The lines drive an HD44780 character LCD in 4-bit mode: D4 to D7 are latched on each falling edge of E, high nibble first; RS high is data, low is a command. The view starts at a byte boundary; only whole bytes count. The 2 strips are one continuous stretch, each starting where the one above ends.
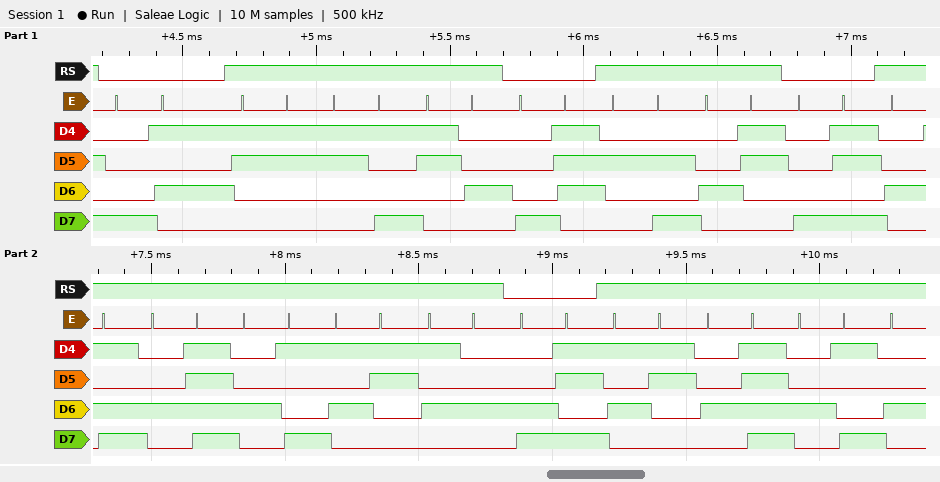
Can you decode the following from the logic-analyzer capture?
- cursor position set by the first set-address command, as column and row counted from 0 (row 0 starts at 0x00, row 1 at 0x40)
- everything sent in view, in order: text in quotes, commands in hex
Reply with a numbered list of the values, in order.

1. column 5, row 0
2. 0x85 "394" 0x87 "*C" 0x8B "MOIST" 0xCB "SOI"
